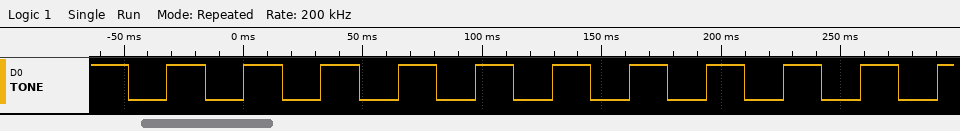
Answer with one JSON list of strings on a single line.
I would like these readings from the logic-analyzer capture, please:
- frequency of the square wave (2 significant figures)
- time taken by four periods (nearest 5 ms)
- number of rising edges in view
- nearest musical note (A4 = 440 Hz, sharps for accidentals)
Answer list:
["31 Hz", "130 ms", "11", "B0"]
